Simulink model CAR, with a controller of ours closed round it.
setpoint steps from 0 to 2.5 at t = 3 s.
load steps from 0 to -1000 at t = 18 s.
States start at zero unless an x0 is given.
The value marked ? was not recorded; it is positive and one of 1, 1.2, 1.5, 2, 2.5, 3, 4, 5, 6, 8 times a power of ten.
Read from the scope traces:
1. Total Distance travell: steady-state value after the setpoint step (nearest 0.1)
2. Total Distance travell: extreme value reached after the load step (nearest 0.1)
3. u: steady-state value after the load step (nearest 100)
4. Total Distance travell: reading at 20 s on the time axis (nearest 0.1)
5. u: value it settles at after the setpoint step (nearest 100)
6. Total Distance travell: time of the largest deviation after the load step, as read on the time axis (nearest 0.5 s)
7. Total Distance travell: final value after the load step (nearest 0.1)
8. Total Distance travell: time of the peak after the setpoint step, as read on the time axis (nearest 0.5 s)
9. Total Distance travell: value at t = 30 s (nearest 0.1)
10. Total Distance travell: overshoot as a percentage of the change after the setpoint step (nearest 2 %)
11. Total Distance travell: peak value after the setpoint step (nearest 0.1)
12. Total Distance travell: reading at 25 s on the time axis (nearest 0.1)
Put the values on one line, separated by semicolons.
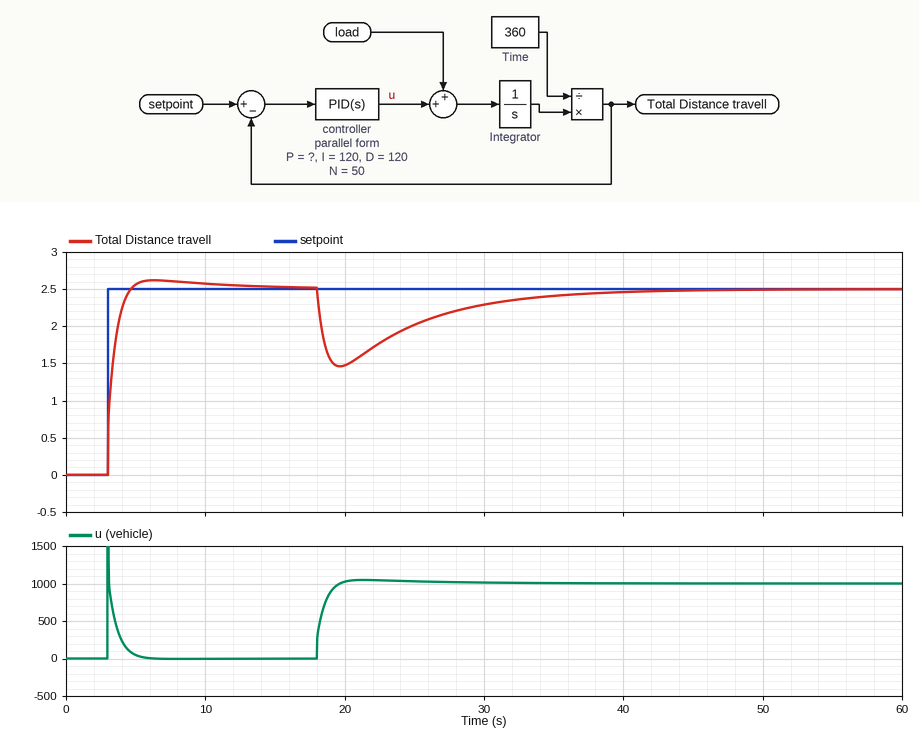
2.5; 1.5; 1000; 1.5; 0; 19.5 s; 2.5; 6.5 s; 2.3; 4 %; 2.6; 2.0
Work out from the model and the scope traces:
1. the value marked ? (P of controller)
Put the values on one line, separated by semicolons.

800
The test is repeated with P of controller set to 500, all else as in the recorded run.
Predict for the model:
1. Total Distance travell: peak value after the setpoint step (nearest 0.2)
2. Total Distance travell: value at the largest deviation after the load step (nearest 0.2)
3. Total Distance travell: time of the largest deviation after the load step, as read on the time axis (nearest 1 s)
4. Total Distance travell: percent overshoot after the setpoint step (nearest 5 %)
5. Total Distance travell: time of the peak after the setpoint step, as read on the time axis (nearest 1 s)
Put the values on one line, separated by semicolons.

2.8; 1.0; 20 s; 10 %; 7 s
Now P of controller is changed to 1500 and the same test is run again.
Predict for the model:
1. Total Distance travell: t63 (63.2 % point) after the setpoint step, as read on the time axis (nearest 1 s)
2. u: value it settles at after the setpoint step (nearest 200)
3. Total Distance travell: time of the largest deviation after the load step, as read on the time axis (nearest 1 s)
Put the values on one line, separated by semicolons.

3 s; 0; 19 s
